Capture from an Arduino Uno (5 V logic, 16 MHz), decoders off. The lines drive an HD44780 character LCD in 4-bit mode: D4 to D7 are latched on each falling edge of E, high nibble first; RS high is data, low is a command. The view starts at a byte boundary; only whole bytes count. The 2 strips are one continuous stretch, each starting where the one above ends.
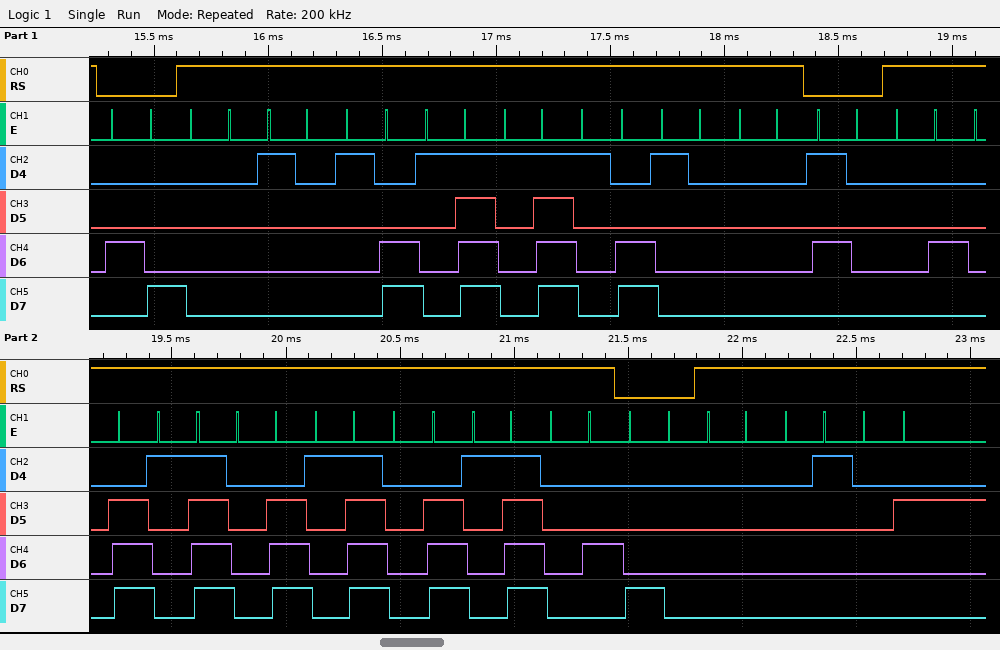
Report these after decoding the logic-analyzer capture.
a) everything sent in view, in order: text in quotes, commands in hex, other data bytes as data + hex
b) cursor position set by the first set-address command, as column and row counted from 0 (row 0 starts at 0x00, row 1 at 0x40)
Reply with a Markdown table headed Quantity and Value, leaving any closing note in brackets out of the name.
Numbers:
| Quantity | Value |
|---|---|
| everything sent in view, in order: text in quotes, commands in hex, other data bytes as data + hex | 0x48 data 00 10 1C 1F 1F 1C 10 00 0x50 data 04 0E 1F 0E 1F 0E 1F 04 0x80 data 00 01 02 |
| cursor position set by the first set-address command, as column and row counted from 0 | column 0, row 0 |
